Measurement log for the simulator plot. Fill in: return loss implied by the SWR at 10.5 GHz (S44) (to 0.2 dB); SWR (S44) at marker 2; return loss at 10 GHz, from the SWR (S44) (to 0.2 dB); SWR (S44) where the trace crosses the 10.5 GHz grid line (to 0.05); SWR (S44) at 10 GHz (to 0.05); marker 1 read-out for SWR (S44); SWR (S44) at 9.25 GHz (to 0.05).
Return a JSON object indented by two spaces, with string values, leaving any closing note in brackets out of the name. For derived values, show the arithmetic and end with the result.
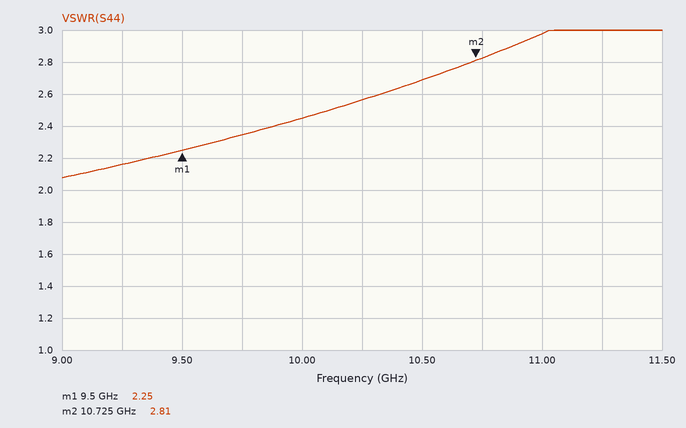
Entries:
{
  "return loss implied by the SWR at 10.5 GHz (S44)": "−20 log10((2.7 − 1)/(2.7 + 1)) ≈ 6.8 dB",
  "SWR (S44) at marker 2": "2.81",
  "return loss at 10 GHz, from the SWR (S44)": "−20 log10((2.45 − 1)/(2.45 + 1)) ≈ 7.53 dB, so 7.6 dB to the nearest 0.2 dB",
  "SWR (S44) where the trace crosses the 10.5 GHz grid line": "2.70",
  "SWR (S44) at 10 GHz": "2.45",
  "marker 1 read-out for SWR": "2.25",
  "SWR (S44) at 9.25 GHz": "2.15"
}
